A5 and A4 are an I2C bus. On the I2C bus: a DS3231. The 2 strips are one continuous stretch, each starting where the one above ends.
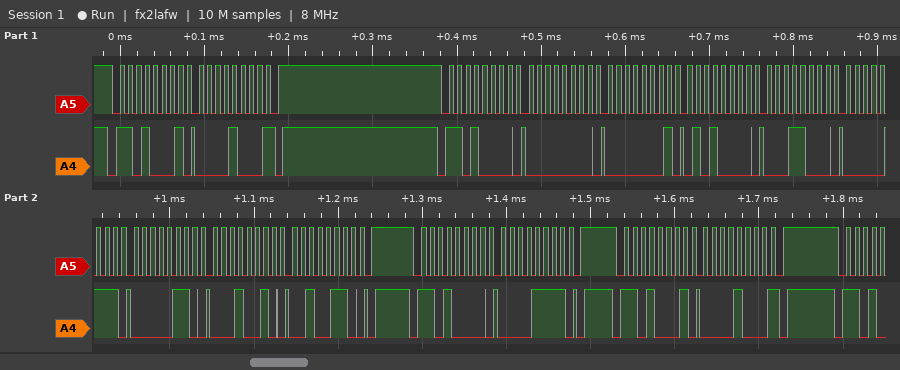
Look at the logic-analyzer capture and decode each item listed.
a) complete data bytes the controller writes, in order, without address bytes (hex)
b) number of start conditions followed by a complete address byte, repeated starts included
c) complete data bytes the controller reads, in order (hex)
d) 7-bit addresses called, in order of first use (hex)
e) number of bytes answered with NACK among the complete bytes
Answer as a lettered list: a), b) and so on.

a) 00 01 50 18 07 06 12 26 0F
b) 4
c) 08 08
d) 0x68
e) 2
